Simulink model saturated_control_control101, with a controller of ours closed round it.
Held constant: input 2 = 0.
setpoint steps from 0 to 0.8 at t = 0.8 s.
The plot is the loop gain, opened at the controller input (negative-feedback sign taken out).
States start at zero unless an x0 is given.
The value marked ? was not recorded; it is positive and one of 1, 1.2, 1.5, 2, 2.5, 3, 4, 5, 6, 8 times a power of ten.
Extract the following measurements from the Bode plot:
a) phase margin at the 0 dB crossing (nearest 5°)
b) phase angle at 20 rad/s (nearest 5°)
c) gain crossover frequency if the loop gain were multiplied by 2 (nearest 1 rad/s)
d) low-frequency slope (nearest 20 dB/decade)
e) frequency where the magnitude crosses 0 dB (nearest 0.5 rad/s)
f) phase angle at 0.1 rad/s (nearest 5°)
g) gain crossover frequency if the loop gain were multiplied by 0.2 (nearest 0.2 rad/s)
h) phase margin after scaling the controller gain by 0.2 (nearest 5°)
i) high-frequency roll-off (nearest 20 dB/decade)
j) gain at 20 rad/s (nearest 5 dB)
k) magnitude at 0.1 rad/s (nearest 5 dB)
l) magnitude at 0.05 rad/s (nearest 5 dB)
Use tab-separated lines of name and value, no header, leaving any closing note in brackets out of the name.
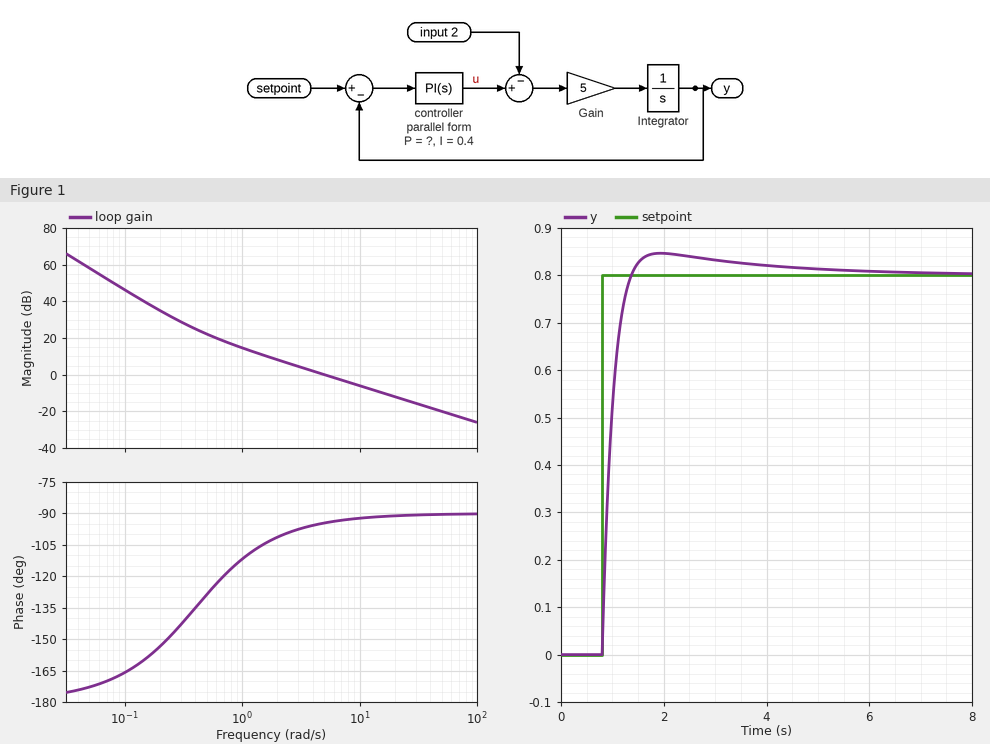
phase margin at the 0 dB crossing	85°
phase angle at 20 rad/s	-90°
gain crossover frequency if the loop gain were multiplied by 2	10 rad/s
low-frequency slope	-40 dB/decade
frequency where the magnitude crosses 0 dB	5.0 rad/s
phase angle at 0.1 rad/s	-165°
gain crossover frequency if the loop gain were multiplied by 0.2	1.0 rad/s
phase margin after scaling the controller gain by 0.2	70°
high-frequency roll-off	-20 dB/decade
gain at 20 rad/s	-10 dB
magnitude at 0.1 rad/s	45 dB
magnitude at 0.05 rad/s	60 dB
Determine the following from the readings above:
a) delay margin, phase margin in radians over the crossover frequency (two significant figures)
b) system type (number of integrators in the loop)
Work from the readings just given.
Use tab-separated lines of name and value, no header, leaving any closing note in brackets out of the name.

delay margin, phase margin in radians over the crossover frequency	0.30 s
system type	2
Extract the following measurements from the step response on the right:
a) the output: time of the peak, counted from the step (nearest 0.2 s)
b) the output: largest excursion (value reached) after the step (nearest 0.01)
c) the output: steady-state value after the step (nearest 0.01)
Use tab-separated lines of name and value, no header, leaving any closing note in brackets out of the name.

the output: time of the peak, counted from the step	1.2 s
the output: largest excursion (value reached) after the step	0.85
the output: steady-state value after the step	0.80
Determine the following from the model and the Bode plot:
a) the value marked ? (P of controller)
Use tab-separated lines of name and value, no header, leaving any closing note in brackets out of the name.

the value marked ?	1
